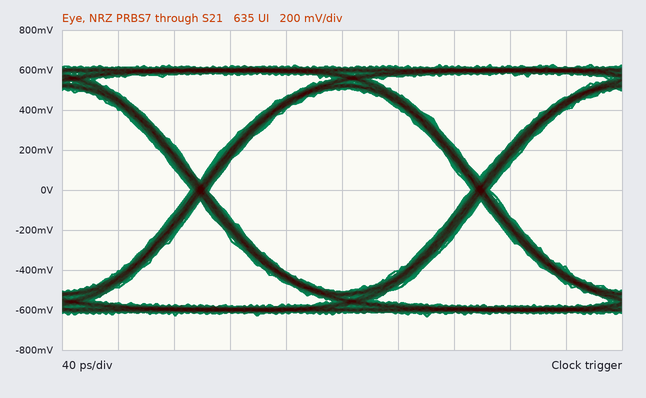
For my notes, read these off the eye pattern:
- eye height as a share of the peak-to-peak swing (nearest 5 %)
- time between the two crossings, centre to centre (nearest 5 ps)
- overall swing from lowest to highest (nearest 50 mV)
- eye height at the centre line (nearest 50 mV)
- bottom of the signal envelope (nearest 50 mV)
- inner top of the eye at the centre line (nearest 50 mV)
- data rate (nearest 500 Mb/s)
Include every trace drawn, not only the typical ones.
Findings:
80 %
200 ps
1.25 V
1.00 V
-650 mV
500 mV
5.0 Gb/s
